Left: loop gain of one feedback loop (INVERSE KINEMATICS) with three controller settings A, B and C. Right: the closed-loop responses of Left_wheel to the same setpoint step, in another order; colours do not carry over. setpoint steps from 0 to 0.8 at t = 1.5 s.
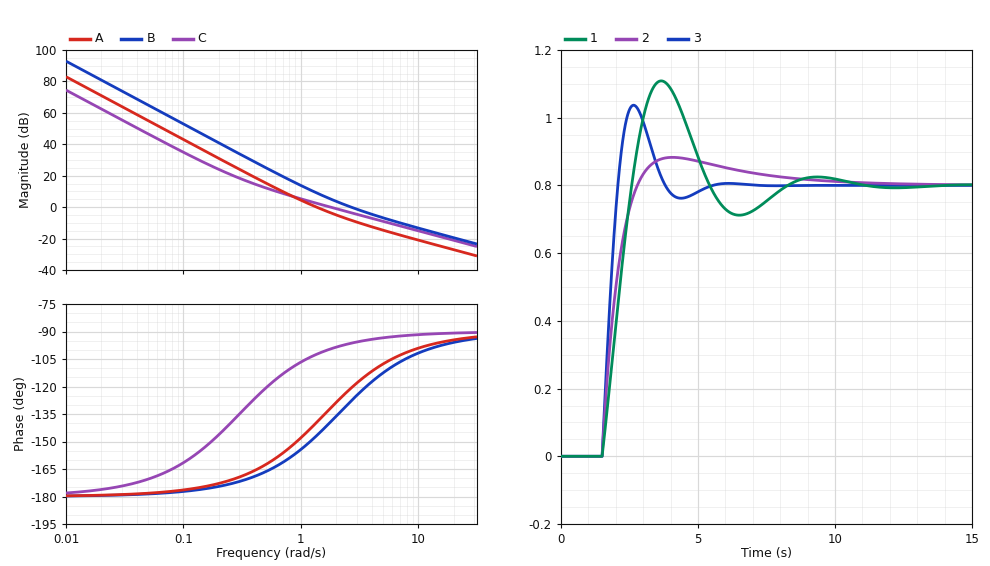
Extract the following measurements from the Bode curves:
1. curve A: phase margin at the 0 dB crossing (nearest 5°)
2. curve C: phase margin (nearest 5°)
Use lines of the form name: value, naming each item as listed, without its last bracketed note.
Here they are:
curve A: phase margin at the 0 dB crossing: 40°
curve C: phase margin: 80°
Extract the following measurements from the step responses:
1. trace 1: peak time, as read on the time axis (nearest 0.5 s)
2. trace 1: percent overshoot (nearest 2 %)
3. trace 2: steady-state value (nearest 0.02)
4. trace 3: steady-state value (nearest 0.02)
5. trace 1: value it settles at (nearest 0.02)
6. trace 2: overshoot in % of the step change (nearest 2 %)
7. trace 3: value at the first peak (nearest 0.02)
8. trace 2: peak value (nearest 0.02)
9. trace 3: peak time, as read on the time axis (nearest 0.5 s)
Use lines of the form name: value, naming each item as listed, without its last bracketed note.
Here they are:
trace 1: peak time, as read on the time axis: 3.5 s
trace 1: percent overshoot: 38 %
trace 2: steady-state value: 0.80
trace 3: steady-state value: 0.80
trace 1: value it settles at: 0.80
trace 2: overshoot in % of the step change: 10 %
trace 3: value at the first peak: 1.04
trace 2: peak value: 0.88
trace 3: peak time, as read on the time axis: 2.5 s
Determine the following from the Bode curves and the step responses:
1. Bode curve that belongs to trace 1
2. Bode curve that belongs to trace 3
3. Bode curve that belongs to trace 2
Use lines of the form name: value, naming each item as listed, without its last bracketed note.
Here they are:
Bode curve that belongs to trace 1: A
Bode curve that belongs to trace 3: B
Bode curve that belongs to trace 2: C
